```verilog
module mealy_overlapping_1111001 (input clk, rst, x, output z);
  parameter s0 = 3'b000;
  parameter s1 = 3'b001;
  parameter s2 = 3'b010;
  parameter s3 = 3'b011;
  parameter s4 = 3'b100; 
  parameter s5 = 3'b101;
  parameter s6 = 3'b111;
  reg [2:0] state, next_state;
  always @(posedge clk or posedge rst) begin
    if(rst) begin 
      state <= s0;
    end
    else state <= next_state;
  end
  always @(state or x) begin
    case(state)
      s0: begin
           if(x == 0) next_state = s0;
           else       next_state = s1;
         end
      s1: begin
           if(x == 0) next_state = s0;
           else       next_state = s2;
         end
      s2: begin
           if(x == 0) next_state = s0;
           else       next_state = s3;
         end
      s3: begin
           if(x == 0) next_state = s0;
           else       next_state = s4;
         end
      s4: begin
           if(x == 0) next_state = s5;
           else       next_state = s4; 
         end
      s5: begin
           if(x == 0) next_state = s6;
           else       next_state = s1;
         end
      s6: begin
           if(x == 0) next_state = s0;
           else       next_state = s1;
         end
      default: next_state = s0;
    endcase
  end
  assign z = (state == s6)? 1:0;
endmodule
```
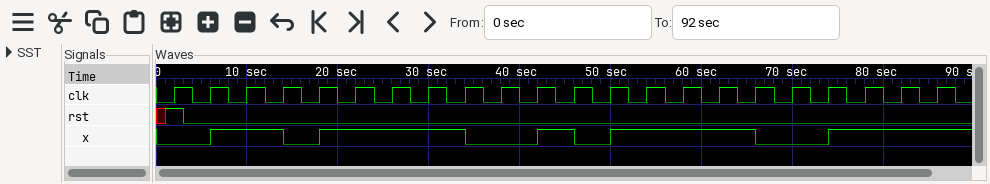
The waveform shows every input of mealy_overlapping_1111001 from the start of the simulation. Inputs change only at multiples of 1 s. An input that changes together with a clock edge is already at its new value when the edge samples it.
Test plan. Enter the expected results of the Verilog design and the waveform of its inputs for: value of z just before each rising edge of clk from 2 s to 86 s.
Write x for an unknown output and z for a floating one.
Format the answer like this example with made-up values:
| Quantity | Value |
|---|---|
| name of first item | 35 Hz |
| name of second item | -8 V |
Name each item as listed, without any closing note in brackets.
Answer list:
| Quantity | Value |
|---|---|
| value of z just before each rising edge of clk from 2 s to 86 s | 0 0 0 0 0 0 0 0 0 0 1 0 0 0 0 0 0 0 1 0 0 0 |
